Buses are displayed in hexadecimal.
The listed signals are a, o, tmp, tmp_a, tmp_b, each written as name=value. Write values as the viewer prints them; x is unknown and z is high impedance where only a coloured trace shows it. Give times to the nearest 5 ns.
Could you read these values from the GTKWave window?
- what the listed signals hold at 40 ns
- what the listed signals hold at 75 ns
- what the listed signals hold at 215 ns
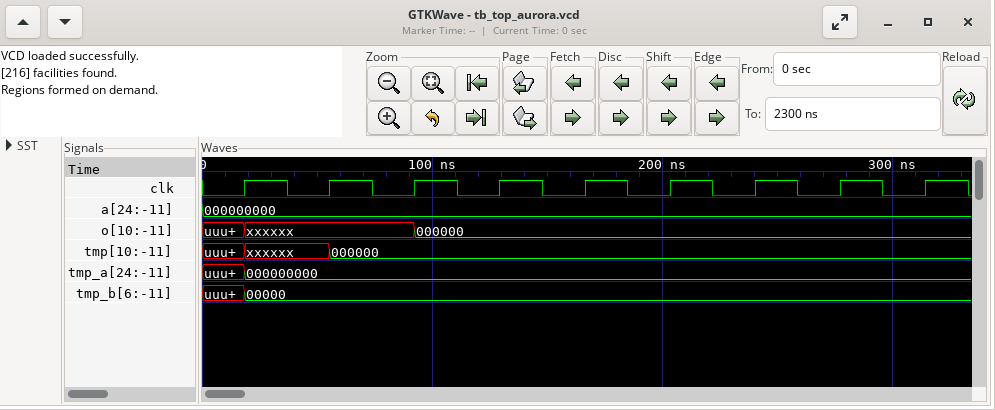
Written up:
a=000000000, o=xxxxxx, tmp=xxxxxx, tmp_a=000000000, tmp_b=00000
a=000000000, o=xxxxxx, tmp=000000, tmp_a=000000000, tmp_b=00000
a=000000000, o=000000, tmp=000000, tmp_a=000000000, tmp_b=00000
